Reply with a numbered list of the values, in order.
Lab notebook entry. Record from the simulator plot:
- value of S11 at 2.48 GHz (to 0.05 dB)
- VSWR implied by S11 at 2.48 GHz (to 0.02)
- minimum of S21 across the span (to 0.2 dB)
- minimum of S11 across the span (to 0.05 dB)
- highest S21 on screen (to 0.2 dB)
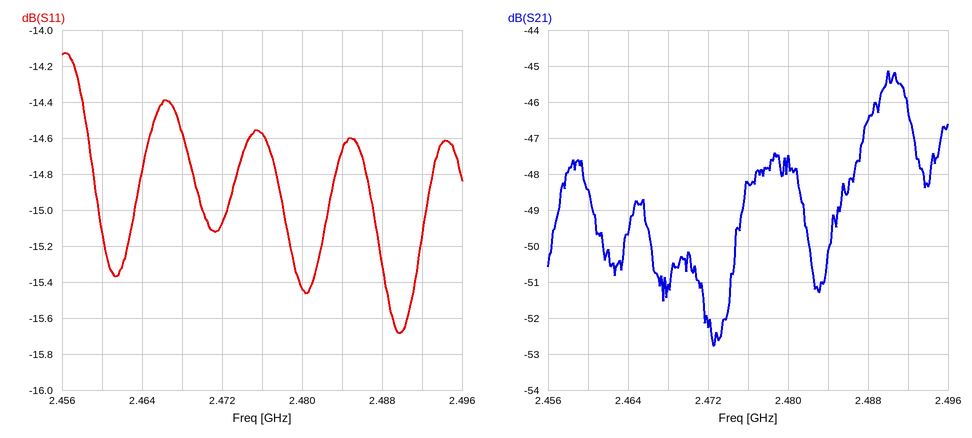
1. -15.45 dB
2. 1.40
3. -52.8 dB
4. -15.70 dB
5. -45.2 dB
